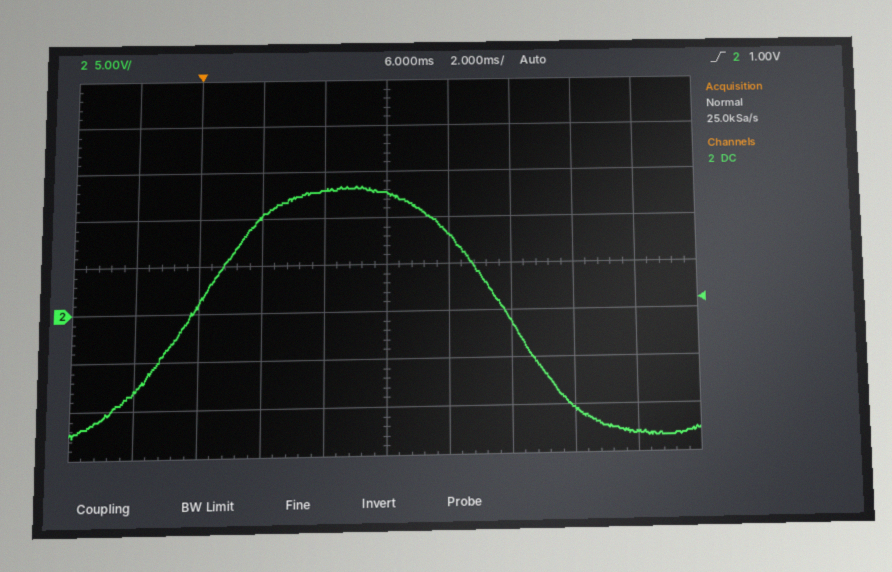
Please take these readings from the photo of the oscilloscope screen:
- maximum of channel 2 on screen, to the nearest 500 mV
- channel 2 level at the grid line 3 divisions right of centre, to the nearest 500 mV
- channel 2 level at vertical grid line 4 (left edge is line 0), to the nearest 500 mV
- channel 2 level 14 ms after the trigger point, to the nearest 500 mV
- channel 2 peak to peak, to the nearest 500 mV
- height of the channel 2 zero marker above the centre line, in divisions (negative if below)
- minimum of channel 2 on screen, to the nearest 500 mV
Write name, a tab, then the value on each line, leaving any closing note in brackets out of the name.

maximum of channel 2 on screen, to the nearest 500 mV	13.5 V
channel 2 level at the grid line 3 divisions right of centre, to the nearest 500 mV	-10.5 V
channel 2 level at vertical grid line 4 (left edge is line 0), to the nearest 500 mV	13.0 V
channel 2 level 14 ms after the trigger point, to the nearest 500 mV	-13.0 V
channel 2 peak to peak, to the nearest 500 mV	26.5 V
height of the channel 2 zero marker above the centre line, in divisions	-1.0 div
minimum of channel 2 on screen, to the nearest 500 mV	-13.0 V
